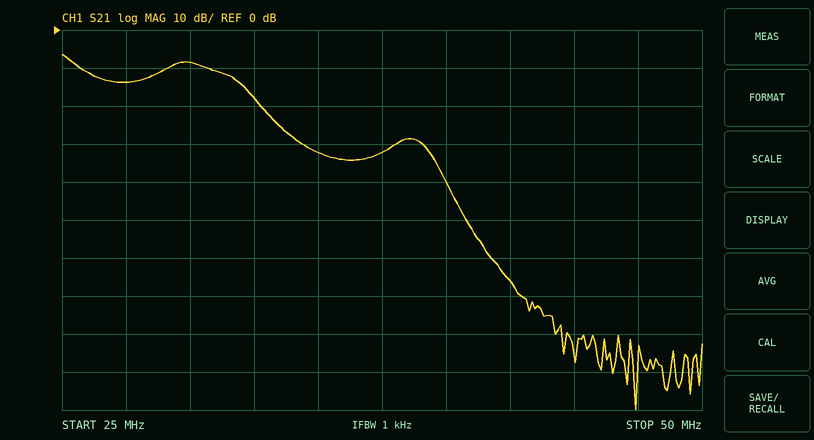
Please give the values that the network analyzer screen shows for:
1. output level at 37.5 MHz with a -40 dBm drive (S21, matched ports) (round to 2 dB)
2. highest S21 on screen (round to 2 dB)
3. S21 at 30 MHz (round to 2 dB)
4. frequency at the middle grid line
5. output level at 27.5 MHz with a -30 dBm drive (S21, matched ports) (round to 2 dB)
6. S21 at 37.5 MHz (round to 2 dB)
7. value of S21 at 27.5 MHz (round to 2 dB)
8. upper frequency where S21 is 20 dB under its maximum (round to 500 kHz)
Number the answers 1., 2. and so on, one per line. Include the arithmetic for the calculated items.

1. -40 dBm + (-32 dB) = -72 dBm
2. -6 dB
3. -8 dB
4. 37.5 MHz
5. -30 dBm + (-14 dB) = -44 dBm
6. -32 dB
7. -14 dB
8. 33.5 MHz
